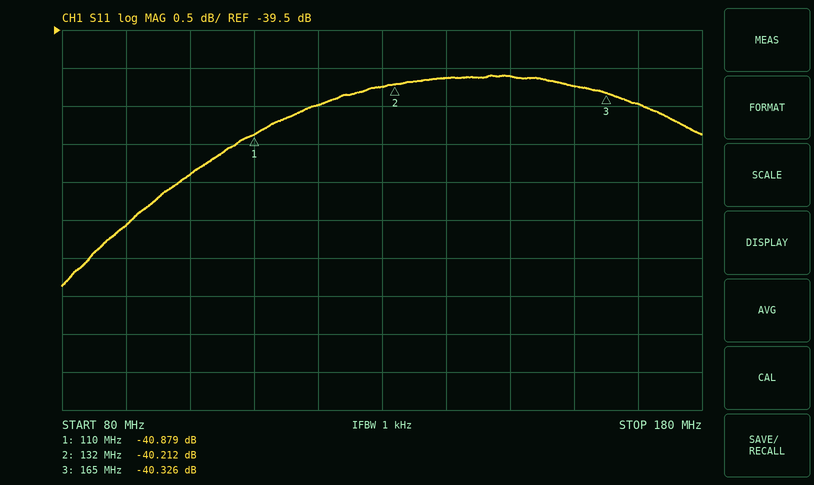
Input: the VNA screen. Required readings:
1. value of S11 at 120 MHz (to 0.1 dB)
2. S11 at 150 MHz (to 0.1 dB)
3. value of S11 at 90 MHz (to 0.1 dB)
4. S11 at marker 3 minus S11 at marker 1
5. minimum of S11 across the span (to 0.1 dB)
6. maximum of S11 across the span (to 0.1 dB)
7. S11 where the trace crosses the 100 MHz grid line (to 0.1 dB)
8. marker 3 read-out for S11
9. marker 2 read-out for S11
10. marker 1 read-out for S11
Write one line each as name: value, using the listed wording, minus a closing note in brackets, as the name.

value of S11 at 120 MHz: -40.5 dB
S11 at 150 MHz: -40.1 dB
value of S11 at 90 MHz: -42.1 dB
S11 at marker 3 minus S11 at marker 1: 0.553 dB
minimum of S11 across the span: -42.9 dB
maximum of S11 across the span: -40.1 dB
S11 where the trace crosses the 100 MHz grid line: -41.4 dB
marker 3 read-out for S11: -40.326 dB
marker 2 read-out for S11: -40.212 dB
marker 1 read-out for S11: -40.879 dB
